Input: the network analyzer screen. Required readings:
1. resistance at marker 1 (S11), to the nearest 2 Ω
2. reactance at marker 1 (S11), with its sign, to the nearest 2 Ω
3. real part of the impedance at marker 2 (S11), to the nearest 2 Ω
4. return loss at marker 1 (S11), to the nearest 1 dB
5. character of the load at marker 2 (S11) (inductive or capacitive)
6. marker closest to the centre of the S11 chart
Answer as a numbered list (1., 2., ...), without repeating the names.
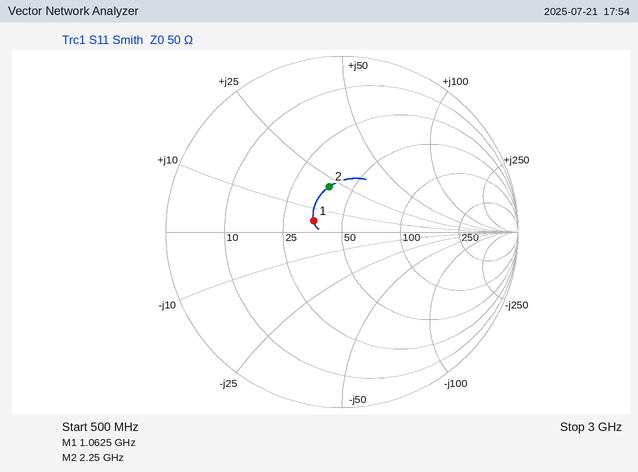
1. 36 Ω
2. +4 Ω
3. 38 Ω
4. 15 dB
5. inductive
6. marker 1
